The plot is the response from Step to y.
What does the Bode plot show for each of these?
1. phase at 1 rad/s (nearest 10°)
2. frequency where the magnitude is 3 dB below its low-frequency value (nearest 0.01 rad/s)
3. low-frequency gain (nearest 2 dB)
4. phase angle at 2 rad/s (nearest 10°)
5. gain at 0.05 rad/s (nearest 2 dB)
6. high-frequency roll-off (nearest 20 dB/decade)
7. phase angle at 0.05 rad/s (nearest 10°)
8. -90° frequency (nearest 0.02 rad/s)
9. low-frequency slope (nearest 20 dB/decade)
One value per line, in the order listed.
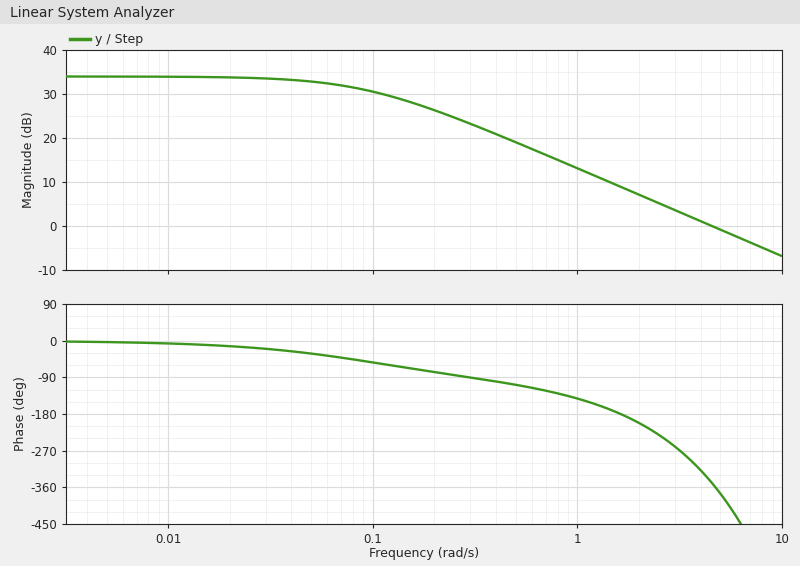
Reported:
-140°
0.09 rad/s
34 dB
-200°
32 dB
-20 dB/decade
-30°
0.30 rad/s
0 dB/decade
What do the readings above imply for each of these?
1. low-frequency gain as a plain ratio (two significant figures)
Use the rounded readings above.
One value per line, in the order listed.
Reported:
50
